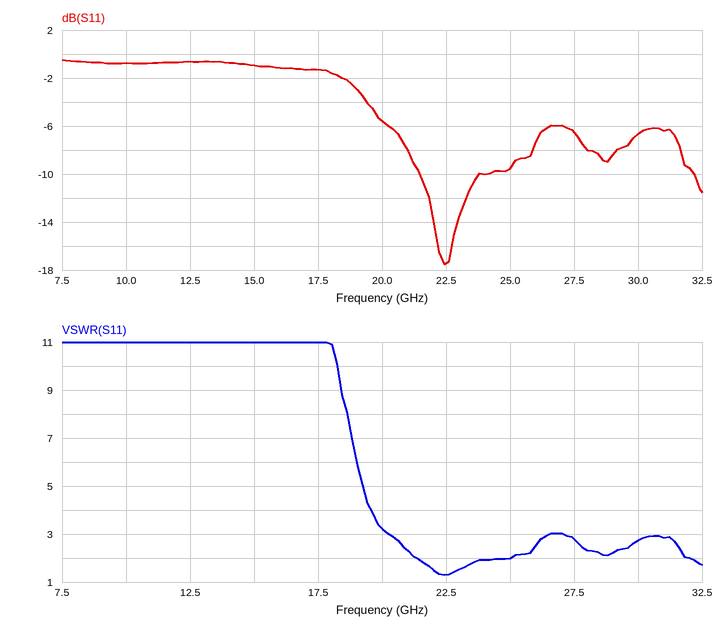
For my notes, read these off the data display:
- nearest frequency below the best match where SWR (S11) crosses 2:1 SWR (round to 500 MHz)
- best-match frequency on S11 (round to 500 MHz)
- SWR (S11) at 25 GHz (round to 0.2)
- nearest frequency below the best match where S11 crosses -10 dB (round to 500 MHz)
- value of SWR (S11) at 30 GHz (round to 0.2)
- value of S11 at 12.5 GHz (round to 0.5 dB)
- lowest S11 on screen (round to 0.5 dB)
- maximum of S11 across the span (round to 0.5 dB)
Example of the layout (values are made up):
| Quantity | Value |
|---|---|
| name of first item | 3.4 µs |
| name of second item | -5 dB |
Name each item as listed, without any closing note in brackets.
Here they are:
| Quantity | Value |
|---|---|
| nearest frequency below the best match where SWR (S11) crosses 2:1 SWR | 21.5 GHz |
| best-match frequency on S11 | 22.5 GHz |
| SWR (S11) at 25 GHz | 2.0 |
| nearest frequency below the best match where S11 crosses -10 dB | 21.5 GHz |
| value of SWR (S11) at 30 GHz | 2.8 |
| value of S11 at 12.5 GHz | -0.5 dB |
| lowest S11 on screen | -17.5 dB |
| maximum of S11 across the span | -0.5 dB |
